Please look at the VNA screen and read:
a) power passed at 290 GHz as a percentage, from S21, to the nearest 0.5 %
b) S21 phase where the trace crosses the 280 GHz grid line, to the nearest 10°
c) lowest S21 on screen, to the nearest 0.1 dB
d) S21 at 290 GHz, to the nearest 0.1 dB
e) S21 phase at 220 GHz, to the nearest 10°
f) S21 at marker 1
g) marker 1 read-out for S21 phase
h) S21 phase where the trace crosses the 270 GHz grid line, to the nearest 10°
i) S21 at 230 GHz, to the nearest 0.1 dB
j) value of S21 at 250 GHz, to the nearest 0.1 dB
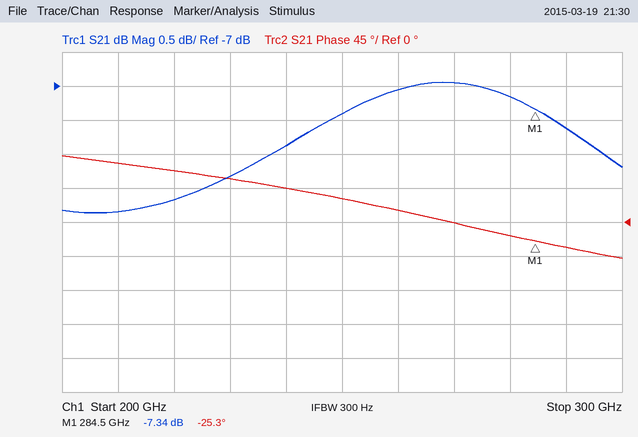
17.5 %
-20°
-8.9 dB
-7.6 dB
70°
-7.34 dB
-25.3°
0°
-8.3 dB
-7.4 dB
